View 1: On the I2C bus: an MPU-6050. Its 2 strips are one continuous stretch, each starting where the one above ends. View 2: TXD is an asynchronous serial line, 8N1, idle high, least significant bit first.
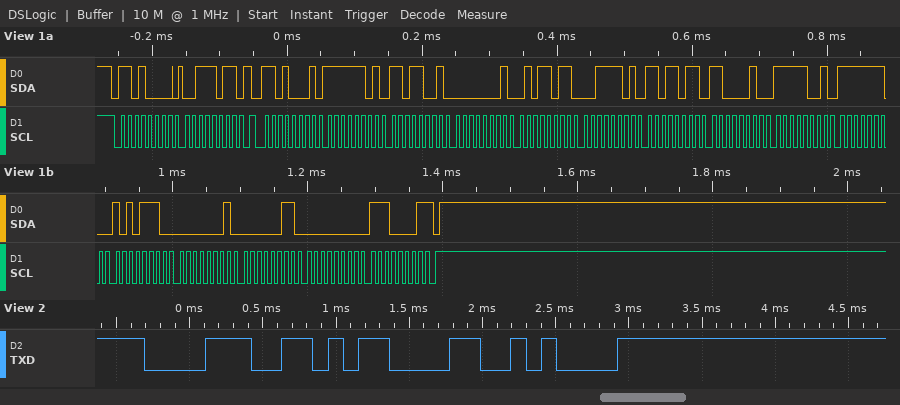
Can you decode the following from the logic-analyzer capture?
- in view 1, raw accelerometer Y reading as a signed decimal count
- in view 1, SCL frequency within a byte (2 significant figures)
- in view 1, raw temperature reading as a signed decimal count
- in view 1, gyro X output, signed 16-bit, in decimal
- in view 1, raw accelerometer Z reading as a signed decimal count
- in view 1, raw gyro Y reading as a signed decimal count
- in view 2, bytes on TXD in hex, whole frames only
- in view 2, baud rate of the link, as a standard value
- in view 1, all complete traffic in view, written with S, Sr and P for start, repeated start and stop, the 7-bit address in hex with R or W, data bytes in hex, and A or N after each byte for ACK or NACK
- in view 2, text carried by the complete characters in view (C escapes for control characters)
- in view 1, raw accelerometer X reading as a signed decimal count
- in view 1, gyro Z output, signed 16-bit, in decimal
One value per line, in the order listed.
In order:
347
100 kHz
-15623
-338
15835
259
38 0D 0A
9600 baud
S 68W A 3B A Sr 68R A FD A D9 A 01 A 5B A 3D A DB A C2 A F9 A FE A AE A 01 A 03 A 00 A E1 N P
"8\r\n"
-551
225
